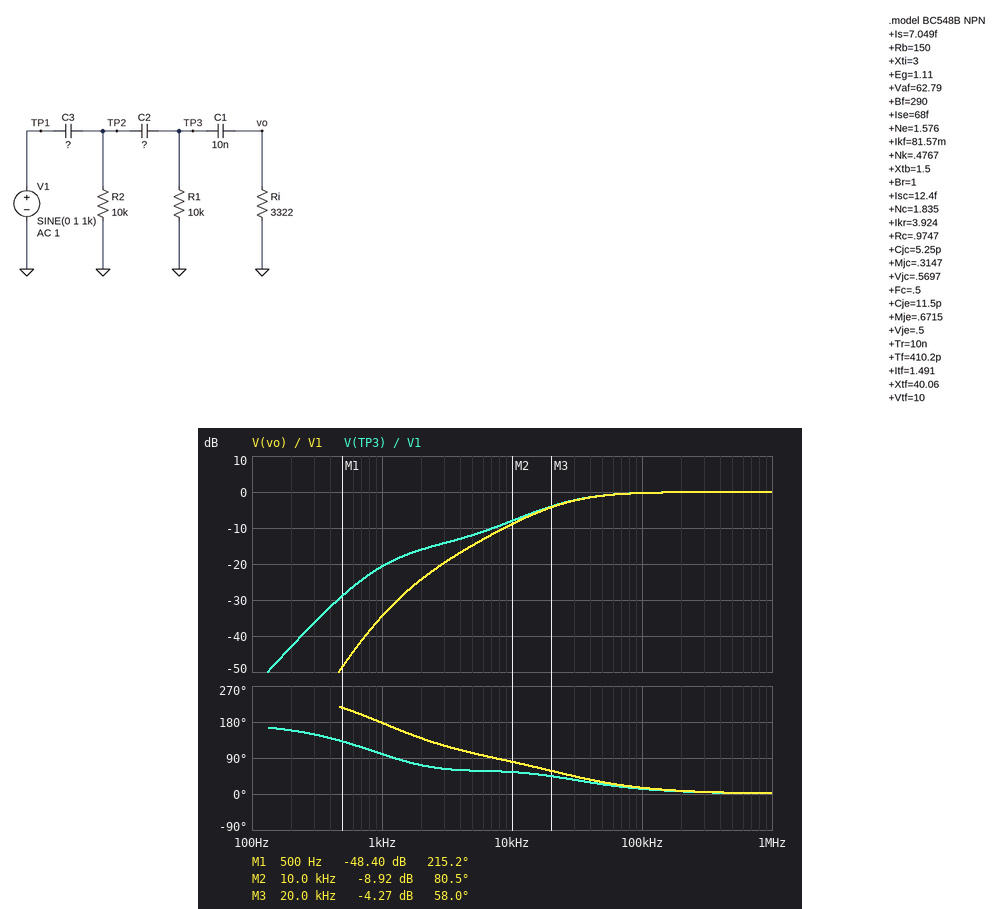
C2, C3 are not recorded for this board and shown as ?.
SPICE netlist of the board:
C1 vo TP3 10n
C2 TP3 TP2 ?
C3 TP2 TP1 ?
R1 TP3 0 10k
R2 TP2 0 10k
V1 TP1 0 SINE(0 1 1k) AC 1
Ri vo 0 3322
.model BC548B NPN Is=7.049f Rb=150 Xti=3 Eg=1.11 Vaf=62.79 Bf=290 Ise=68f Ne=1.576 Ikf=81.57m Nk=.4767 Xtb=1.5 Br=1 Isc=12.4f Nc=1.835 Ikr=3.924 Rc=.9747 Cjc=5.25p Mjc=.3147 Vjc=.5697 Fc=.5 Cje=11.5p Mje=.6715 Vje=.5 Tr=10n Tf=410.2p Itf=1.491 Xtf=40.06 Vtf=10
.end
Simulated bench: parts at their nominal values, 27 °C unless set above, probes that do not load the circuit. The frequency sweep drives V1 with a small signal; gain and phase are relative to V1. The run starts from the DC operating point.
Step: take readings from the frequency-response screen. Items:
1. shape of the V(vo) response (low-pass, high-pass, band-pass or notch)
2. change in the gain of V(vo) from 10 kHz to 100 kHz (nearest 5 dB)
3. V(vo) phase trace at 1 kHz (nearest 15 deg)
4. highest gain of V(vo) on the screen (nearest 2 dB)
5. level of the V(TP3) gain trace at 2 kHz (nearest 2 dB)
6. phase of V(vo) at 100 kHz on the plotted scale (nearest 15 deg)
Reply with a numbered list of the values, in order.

1. high-pass
2. 10 dB
3. 180 deg
4. 0 dB
5. -16 dB
6. 15 deg
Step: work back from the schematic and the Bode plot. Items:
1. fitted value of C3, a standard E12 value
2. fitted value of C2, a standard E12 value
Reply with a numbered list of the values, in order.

1. 12 nF
2. 3.9 nF
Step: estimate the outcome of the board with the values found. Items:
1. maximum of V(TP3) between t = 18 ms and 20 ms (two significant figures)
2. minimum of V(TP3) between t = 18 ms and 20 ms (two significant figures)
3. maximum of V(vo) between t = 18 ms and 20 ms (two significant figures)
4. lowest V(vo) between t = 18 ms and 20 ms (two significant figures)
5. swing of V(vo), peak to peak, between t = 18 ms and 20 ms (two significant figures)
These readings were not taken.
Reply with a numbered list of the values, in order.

1. 92 mV
2. -92 mV
3. 19 mV
4. -19 mV
5. 38 mV
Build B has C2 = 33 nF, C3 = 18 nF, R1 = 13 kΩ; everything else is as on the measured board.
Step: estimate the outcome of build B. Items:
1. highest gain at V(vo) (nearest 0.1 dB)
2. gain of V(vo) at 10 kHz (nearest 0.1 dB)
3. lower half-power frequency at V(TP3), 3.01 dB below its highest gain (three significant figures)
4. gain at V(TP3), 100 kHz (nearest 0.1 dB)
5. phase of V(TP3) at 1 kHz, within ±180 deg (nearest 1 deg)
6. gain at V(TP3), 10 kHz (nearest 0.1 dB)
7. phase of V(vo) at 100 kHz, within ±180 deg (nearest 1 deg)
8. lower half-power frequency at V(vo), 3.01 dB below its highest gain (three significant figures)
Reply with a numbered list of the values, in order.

1. 0 dB
2. -2.9 dB
3. 7.17 kHz
4. 0 dB
5. 59 deg
6. -2.0 dB
7. 6 deg
8. 9.83 kHz
